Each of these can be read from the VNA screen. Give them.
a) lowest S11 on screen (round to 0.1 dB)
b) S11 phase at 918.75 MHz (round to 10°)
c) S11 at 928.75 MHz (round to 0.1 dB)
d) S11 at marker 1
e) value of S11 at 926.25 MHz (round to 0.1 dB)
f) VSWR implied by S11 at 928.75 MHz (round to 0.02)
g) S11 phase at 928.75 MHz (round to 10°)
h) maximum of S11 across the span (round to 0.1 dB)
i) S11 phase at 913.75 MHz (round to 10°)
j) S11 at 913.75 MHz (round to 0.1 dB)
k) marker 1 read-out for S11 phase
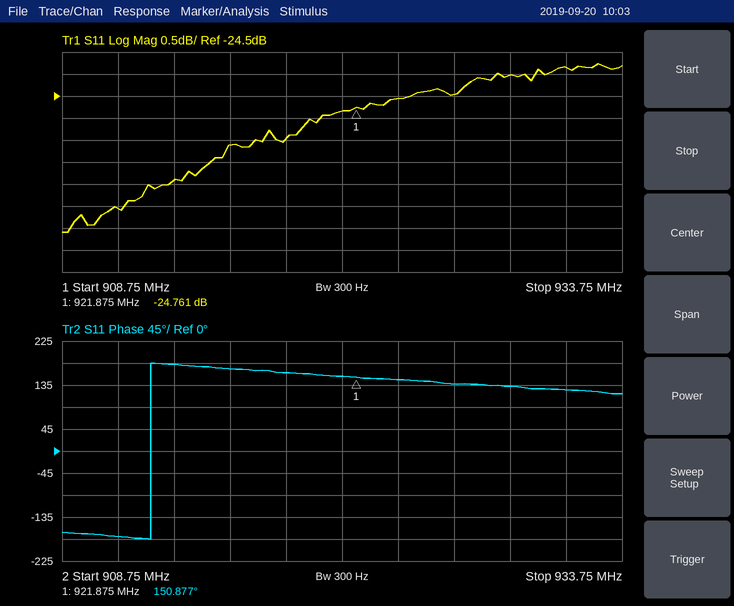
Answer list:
-27.6 dB
160°
-24.0 dB
-24.761 dB
-24.5 dB
1.14
130°
-23.8 dB
180°
-26.4 dB
150.877°
